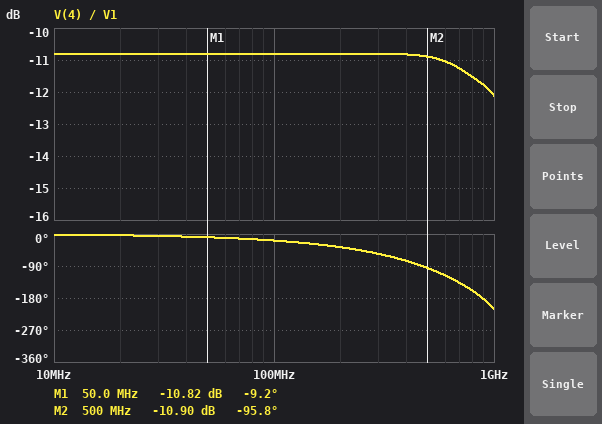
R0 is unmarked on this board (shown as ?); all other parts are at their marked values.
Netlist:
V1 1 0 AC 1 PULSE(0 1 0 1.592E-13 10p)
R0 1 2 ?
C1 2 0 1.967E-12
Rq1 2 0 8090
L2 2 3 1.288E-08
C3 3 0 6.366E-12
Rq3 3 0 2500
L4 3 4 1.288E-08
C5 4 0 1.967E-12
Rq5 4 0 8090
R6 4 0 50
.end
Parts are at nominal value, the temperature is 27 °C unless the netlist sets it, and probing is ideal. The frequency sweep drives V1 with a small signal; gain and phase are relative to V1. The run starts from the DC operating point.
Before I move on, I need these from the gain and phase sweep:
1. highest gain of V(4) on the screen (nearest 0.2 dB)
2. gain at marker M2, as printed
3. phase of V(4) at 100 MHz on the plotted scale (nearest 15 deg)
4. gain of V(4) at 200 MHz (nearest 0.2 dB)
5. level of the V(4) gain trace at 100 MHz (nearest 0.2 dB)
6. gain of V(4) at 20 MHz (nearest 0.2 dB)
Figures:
-10.8 dB
-10.90 dB
-15 deg
-10.8 dB
-10.8 dB
-10.8 dB
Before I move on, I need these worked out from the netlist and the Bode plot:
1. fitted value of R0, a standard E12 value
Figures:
120 Ω
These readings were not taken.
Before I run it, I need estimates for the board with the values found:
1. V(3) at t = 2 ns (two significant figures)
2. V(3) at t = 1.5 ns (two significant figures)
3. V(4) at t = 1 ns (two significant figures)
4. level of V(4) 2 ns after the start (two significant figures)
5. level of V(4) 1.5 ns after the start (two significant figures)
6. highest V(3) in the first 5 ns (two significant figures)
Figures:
280 mV
300 mV
320 mV
290 mV
280 mV
360 mV
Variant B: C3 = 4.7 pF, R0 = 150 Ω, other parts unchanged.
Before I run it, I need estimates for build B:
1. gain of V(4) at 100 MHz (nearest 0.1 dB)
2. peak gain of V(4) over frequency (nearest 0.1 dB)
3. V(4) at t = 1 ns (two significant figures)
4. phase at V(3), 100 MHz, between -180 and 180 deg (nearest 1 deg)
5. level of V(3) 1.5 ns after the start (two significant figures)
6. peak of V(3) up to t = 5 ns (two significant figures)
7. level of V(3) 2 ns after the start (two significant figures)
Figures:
-12.2 dB
-11.7 dB
280 mV
-7 deg
260 mV
340 mV
240 mV
